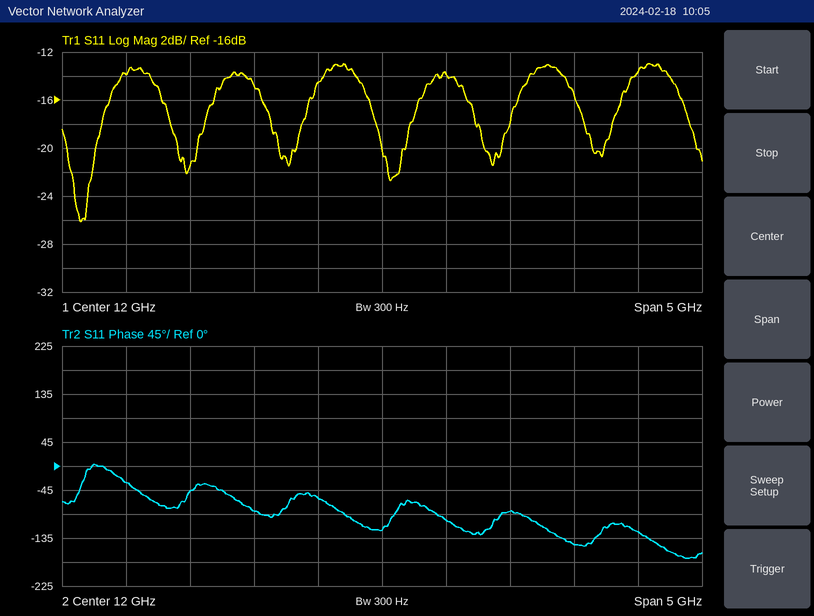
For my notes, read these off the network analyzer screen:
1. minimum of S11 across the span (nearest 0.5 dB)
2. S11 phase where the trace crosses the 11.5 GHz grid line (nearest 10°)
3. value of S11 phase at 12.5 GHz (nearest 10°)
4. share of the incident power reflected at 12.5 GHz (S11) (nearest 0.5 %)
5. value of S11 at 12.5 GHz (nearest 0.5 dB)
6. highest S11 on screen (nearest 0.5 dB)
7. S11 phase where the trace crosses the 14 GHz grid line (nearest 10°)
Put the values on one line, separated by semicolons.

-26.0 dB; -60°; -100°; 4.0 %; -14.0 dB; -13.0 dB; -120°
